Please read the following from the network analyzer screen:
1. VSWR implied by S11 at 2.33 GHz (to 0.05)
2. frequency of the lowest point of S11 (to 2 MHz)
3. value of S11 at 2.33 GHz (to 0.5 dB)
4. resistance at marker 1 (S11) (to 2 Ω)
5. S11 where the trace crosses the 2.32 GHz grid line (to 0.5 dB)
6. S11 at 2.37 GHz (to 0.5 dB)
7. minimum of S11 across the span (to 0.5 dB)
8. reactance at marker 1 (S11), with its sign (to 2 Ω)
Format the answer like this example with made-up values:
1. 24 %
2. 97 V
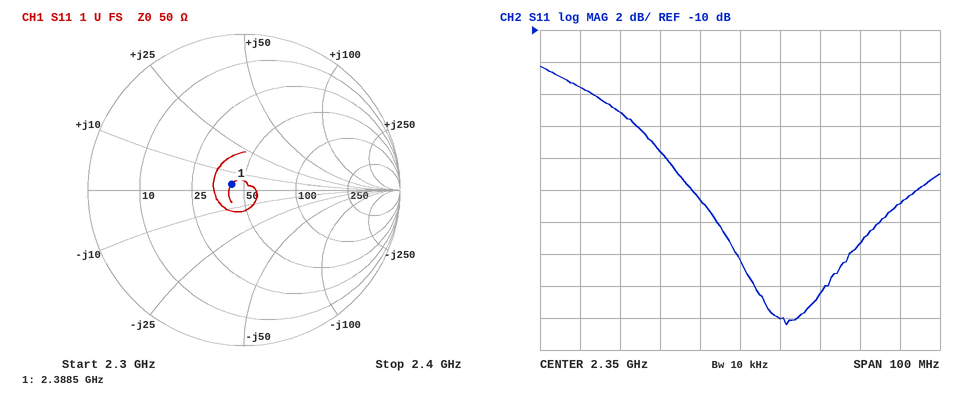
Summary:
1. 1.30
2. 2.362 GHz
3. -17.5 dB
4. 42 Ω
5. -15.0 dB
6. -26.5 dB
7. -28.5 dB
8. +4 Ω
